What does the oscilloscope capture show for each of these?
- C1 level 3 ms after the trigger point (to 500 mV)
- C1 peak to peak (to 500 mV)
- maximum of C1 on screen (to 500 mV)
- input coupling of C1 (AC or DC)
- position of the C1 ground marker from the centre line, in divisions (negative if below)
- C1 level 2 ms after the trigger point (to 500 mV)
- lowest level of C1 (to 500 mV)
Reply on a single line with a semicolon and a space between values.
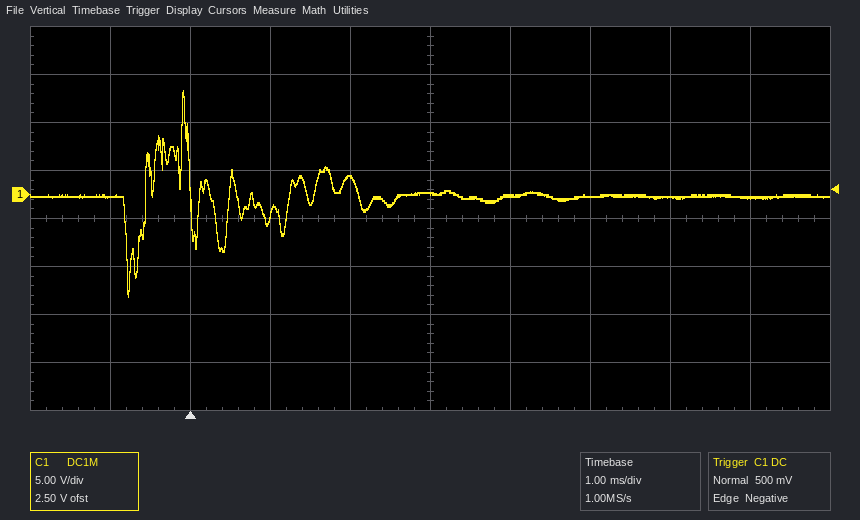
0.0 V; 21.5 V; 11.0 V; DC; +0.5 div; 1.5 V; -10.5 V
